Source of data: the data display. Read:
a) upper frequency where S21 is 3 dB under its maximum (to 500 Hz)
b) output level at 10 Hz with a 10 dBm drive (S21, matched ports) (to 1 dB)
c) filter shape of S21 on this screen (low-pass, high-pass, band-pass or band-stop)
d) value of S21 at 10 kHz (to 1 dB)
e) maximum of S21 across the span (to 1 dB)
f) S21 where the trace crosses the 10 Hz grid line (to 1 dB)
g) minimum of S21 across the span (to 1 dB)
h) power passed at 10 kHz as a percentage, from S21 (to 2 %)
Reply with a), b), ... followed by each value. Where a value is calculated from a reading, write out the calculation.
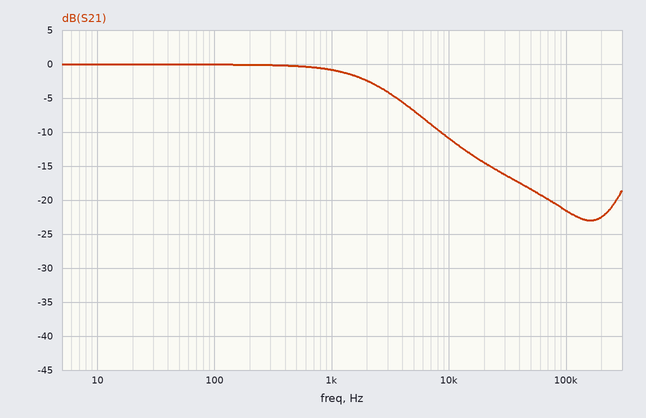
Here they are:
a) 2.5 kHz
b) 10 dBm + (0 dB) = 10 dBm
c) low-pass
d) -11 dB
e) 0 dB
f) 0 dB
g) -23 dB
h) 10^(-11/10) ≈ 8 %
